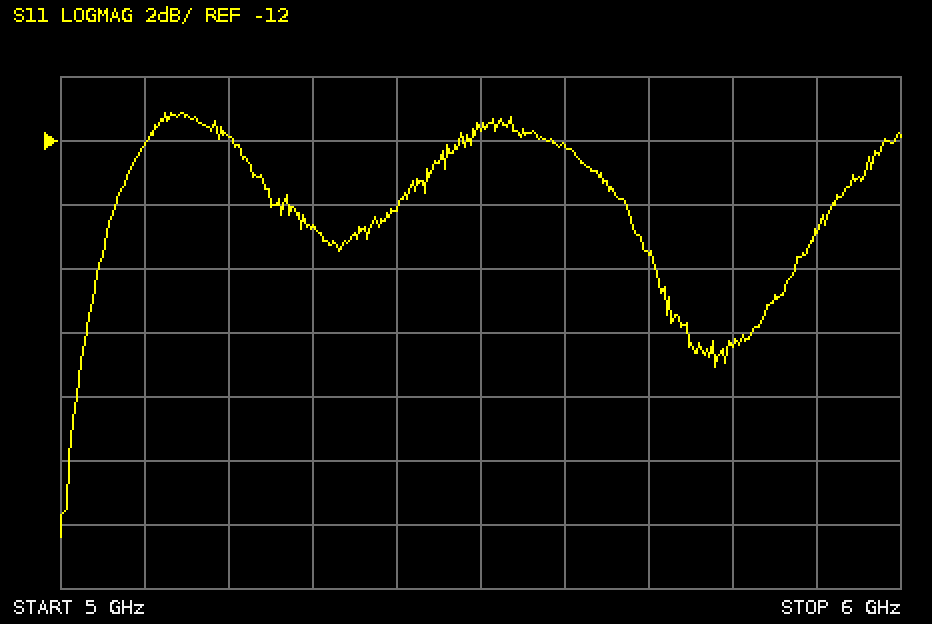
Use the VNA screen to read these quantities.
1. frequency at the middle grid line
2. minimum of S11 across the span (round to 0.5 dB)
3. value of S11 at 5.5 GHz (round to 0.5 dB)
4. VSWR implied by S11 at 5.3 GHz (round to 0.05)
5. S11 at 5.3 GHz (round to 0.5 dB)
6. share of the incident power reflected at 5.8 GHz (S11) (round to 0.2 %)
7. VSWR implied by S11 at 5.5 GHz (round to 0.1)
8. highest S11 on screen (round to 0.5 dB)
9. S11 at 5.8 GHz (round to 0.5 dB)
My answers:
5.5 GHz
-24.5 dB
-11.5 dB
1.45
-14.5 dB
1.4 %
1.7
-11.0 dB
-18.5 dB
